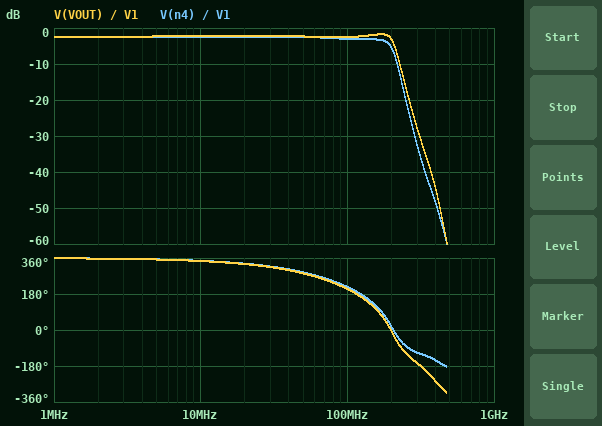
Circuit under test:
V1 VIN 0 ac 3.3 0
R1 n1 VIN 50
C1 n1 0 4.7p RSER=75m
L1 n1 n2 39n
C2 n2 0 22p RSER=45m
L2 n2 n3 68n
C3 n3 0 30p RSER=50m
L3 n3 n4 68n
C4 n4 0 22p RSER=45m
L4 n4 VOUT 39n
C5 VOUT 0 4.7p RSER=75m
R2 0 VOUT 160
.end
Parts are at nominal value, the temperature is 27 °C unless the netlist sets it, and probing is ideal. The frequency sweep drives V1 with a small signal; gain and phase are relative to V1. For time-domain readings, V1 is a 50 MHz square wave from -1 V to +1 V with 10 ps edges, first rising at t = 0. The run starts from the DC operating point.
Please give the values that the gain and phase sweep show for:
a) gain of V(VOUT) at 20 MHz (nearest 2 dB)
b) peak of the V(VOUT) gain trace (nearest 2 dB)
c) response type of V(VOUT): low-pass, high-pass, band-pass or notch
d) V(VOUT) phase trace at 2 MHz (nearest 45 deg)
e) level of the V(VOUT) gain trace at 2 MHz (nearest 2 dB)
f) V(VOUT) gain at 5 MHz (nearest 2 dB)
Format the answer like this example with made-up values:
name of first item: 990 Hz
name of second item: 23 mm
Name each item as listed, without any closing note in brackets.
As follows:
gain of V(VOUT) at 20 MHz: -2 dB
peak of the V(VOUT) gain trace: -2 dB
response type of V(VOUT): low-pass, high-pass, band-pass or notch: low-pass
V(VOUT) phase trace at 2 MHz: 360 deg
level of the V(VOUT) gain trace at 2 MHz: -2 dB
V(VOUT) gain at 5 MHz: -2 dB
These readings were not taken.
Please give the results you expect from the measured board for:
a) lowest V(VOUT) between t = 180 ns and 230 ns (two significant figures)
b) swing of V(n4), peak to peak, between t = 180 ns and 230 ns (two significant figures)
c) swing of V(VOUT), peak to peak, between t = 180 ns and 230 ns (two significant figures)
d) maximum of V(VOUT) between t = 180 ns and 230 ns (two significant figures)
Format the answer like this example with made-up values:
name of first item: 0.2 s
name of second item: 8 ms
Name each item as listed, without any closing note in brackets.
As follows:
lowest V(VOUT) between t = 180 ns and 230 ns: -1.0 V
swing of V(n4), peak to peak, between t = 180 ns and 230 ns: 1.9 V
swing of V(VOUT), peak to peak, between t = 180 ns and 230 ns: 2.0 V
maximum of V(VOUT) between t = 180 ns and 230 ns: 1.0 V
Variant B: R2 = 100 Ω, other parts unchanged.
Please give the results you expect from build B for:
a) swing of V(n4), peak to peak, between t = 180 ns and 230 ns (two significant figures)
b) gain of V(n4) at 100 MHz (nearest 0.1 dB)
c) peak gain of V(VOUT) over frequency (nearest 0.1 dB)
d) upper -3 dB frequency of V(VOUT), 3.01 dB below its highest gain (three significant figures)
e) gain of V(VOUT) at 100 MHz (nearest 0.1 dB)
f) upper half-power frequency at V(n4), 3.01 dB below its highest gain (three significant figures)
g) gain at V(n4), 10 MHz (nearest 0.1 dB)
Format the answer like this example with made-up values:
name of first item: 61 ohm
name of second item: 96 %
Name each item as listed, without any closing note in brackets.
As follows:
swing of V(n4), peak to peak, between t = 180 ns and 230 ns: 1.7 V
gain of V(n4) at 100 MHz: -4.0 dB
peak gain of V(VOUT) over frequency: -3.2 dB
upper -3 dB frequency of V(VOUT), 3.01 dB below its highest gain: 212 MHz
gain of V(VOUT) at 100 MHz: -3.6 dB
upper half-power frequency at V(n4), 3.01 dB below its highest gain: 207 MHz
gain at V(n4), 10 MHz: -3.5 dB
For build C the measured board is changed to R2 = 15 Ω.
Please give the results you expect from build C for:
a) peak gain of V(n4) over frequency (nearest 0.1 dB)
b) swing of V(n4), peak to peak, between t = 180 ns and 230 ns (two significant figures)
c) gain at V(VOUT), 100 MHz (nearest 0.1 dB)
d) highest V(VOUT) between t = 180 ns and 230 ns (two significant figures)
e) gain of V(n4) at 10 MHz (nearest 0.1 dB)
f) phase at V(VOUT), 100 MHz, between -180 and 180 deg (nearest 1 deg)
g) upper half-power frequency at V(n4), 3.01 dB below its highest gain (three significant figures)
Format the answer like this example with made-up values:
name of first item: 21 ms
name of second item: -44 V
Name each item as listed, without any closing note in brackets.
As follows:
peak gain of V(n4) over frequency: -1.3 dB
swing of V(n4), peak to peak, between t = 180 ns and 230 ns: 1.2 V
gain at V(VOUT), 100 MHz: -12.7 dB
highest V(VOUT) between t = 180 ns and 230 ns: 310 mV
gain of V(n4) at 10 MHz: -12.6 dB
phase at V(VOUT), 100 MHz, between -180 and 180 deg: -158 deg
upper half-power frequency at V(n4), 3.01 dB below its highest gain: 242 MHz
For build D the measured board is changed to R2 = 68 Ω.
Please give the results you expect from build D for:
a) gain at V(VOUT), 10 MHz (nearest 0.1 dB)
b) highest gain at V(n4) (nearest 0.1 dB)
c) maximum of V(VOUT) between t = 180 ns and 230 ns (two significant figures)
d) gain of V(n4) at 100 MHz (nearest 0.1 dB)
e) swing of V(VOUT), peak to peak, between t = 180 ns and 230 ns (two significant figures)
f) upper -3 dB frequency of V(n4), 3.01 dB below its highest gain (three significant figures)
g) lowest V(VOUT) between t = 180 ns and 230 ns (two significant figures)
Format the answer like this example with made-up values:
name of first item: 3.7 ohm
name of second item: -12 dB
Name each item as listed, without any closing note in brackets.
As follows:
gain at V(VOUT), 10 MHz: -4.8 dB
highest gain at V(n4): -4.7 dB
maximum of V(VOUT) between t = 180 ns and 230 ns: 760 mV
gain of V(n4) at 100 MHz: -4.9 dB
swing of V(VOUT), peak to peak, between t = 180 ns and 230 ns: 1.5 V
upper -3 dB frequency of V(n4), 3.01 dB below its highest gain: 217 MHz
lowest V(VOUT) between t = 180 ns and 230 ns: -760 mV
